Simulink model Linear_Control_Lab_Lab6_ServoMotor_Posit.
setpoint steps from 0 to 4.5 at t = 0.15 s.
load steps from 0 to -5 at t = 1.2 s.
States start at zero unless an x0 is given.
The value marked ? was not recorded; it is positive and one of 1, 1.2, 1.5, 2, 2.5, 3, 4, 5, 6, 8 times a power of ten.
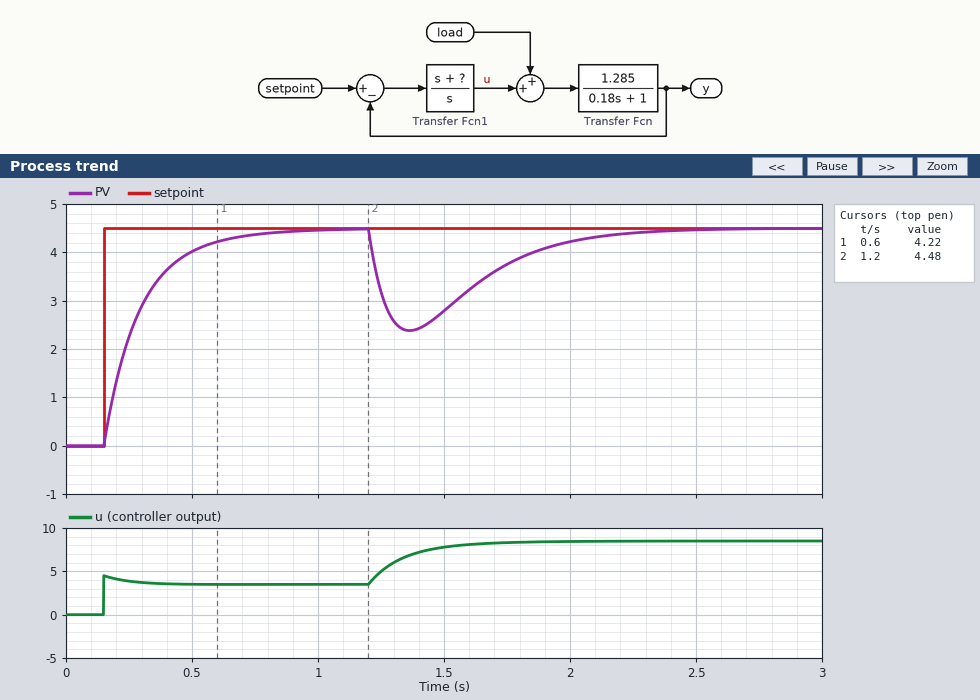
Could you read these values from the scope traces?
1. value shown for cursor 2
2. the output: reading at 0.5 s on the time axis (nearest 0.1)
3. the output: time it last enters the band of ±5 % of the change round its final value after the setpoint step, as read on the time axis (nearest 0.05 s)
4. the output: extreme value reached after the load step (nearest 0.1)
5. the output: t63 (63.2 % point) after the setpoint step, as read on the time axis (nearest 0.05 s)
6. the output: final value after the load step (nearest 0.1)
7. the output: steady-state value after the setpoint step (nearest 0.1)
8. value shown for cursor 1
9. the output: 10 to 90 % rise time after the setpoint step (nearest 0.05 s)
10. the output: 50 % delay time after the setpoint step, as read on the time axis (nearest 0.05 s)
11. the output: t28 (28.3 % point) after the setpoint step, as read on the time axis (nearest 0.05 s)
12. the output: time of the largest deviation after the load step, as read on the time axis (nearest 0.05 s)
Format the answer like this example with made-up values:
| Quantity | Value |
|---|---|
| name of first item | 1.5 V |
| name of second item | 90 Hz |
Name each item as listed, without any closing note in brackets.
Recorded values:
| Quantity | Value |
|---|---|
| value shown for cursor 2 | 4.48 |
| the output: reading at 0.5 s on the time axis | 4.0 |
| the output: time it last enters the band of ±5 % of the change round its final value after the setpoint step, as read on the time axis | 0.65 s |
| the output: extreme value reached after the load step | 2.4 |
| the output: t63 (63.2 % point) after the setpoint step, as read on the time axis | 0.30 s |
| the output: final value after the load step | 4.5 |
| the output: steady-state value after the setpoint step | 4.5 |
| value shown for cursor 1 | 4.22 |
| the output: 10 to 90 % rise time after the setpoint step | 0.35 s |
| the output: 50 % delay time after the setpoint step, as read on the time axis | 0.25 s |
| the output: t28 (28.3 % point) after the setpoint step, as read on the time axis | 0.20 s |
| the output: time of the largest deviation after the load step, as read on the time axis | 1.35 s |
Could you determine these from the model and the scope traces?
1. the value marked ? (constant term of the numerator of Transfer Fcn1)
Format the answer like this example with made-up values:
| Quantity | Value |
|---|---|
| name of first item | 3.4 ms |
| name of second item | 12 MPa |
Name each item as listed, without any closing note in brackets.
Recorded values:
| Quantity | Value |
|---|---|
| the value marked ? | 5 |
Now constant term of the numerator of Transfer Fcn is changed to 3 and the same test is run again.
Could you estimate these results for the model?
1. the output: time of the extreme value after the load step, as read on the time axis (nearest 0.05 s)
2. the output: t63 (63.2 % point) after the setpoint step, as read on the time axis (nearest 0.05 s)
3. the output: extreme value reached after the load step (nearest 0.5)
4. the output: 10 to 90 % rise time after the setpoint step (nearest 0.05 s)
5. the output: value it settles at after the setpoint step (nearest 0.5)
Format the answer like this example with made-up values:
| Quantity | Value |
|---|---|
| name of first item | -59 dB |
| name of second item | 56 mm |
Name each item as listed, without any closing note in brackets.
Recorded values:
| Quantity | Value |
|---|---|
| the output: time of the extreme value after the load step, as read on the time axis | 1.30 s |
| the output: t63 (63.2 % point) after the setpoint step, as read on the time axis | 0.20 s |
| the output: extreme value reached after the load step | 1.5 |
| the output: 10 to 90 % rise time after the setpoint step | 0.15 s |
| the output: value it settles at after the setpoint step | 4.5 |
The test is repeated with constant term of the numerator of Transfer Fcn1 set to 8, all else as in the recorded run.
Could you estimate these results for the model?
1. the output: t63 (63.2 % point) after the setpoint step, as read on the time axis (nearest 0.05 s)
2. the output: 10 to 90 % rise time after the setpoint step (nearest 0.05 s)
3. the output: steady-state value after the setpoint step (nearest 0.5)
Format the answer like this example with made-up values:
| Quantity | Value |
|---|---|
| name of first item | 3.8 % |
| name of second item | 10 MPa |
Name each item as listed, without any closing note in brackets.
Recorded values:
| Quantity | Value |
|---|---|
| the output: t63 (63.2 % point) after the setpoint step, as read on the time axis | 0.25 s |
| the output: 10 to 90 % rise time after the setpoint step | 0.20 s |
| the output: steady-state value after the setpoint step | 4.5 |
